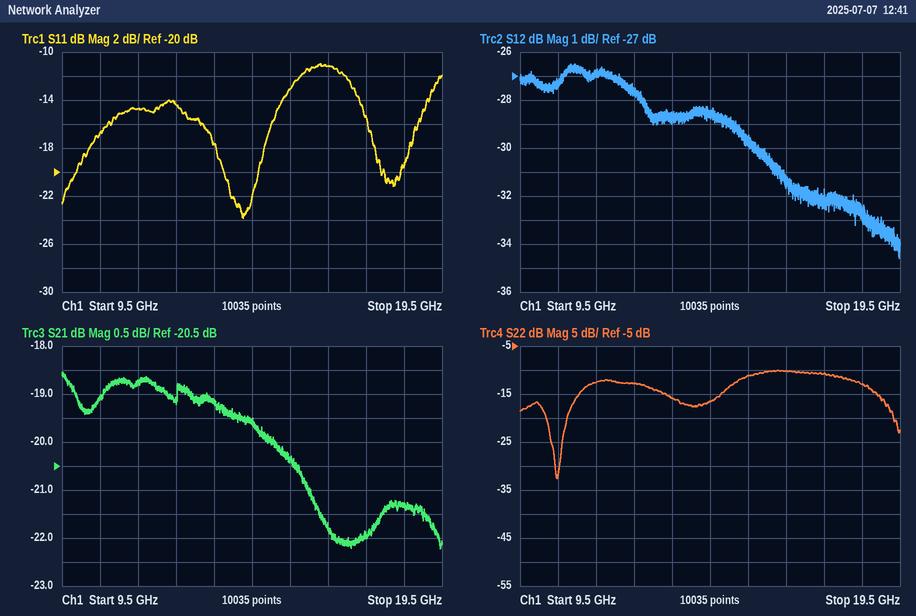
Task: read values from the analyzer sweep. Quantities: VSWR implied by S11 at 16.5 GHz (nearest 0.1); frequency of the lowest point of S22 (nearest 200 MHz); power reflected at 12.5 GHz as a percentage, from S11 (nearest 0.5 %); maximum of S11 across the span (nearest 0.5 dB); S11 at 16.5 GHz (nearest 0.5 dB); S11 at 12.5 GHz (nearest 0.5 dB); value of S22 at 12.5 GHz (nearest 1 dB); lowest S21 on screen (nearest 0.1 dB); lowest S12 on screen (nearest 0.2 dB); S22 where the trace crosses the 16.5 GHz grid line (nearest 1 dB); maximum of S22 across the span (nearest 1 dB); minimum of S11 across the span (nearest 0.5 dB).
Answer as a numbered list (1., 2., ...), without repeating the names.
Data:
1. 1.8
2. 10.4 GHz
3. 3.5 %
4. -11.0 dB
5. -11.0 dB
6. -14.5 dB
7. -13 dB
8. -22.2 dB
9. -34.6 dB
10. -10 dB
11. -10 dB
12. -24.0 dB
